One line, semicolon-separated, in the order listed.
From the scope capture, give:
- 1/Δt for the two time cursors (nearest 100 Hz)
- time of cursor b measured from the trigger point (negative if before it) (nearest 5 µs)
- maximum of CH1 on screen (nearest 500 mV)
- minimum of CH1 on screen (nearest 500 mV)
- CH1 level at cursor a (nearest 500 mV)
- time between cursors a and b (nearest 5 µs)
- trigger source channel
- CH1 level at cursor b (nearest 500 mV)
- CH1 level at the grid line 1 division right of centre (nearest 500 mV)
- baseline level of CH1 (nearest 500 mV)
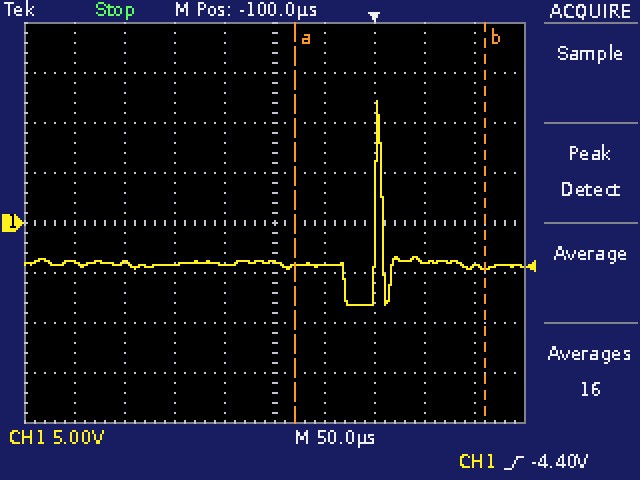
5.3 kHz; +110 µs; 12.0 V; -8.0 V; -4.5 V; 190 µs; CH1; -4.5 V; -4.0 V; -4.0 V
